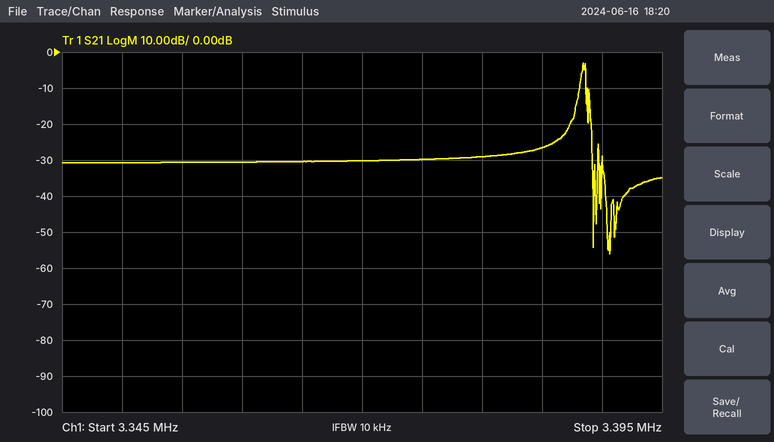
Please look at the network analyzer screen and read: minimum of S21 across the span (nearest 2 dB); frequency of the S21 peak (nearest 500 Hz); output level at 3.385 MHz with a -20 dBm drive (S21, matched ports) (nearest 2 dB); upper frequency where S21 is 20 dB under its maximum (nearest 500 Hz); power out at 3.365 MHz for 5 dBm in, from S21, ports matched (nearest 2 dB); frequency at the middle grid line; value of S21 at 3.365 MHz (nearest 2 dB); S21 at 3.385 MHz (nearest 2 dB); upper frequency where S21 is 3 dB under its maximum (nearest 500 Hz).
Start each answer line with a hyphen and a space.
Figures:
- -56 dB
- 3.3885 MHz
- -46 dBm
- 3.3890 MHz
- -26 dBm
- 3.37 MHz
- -30 dB
- -26 dB
- 3.3885 MHz
